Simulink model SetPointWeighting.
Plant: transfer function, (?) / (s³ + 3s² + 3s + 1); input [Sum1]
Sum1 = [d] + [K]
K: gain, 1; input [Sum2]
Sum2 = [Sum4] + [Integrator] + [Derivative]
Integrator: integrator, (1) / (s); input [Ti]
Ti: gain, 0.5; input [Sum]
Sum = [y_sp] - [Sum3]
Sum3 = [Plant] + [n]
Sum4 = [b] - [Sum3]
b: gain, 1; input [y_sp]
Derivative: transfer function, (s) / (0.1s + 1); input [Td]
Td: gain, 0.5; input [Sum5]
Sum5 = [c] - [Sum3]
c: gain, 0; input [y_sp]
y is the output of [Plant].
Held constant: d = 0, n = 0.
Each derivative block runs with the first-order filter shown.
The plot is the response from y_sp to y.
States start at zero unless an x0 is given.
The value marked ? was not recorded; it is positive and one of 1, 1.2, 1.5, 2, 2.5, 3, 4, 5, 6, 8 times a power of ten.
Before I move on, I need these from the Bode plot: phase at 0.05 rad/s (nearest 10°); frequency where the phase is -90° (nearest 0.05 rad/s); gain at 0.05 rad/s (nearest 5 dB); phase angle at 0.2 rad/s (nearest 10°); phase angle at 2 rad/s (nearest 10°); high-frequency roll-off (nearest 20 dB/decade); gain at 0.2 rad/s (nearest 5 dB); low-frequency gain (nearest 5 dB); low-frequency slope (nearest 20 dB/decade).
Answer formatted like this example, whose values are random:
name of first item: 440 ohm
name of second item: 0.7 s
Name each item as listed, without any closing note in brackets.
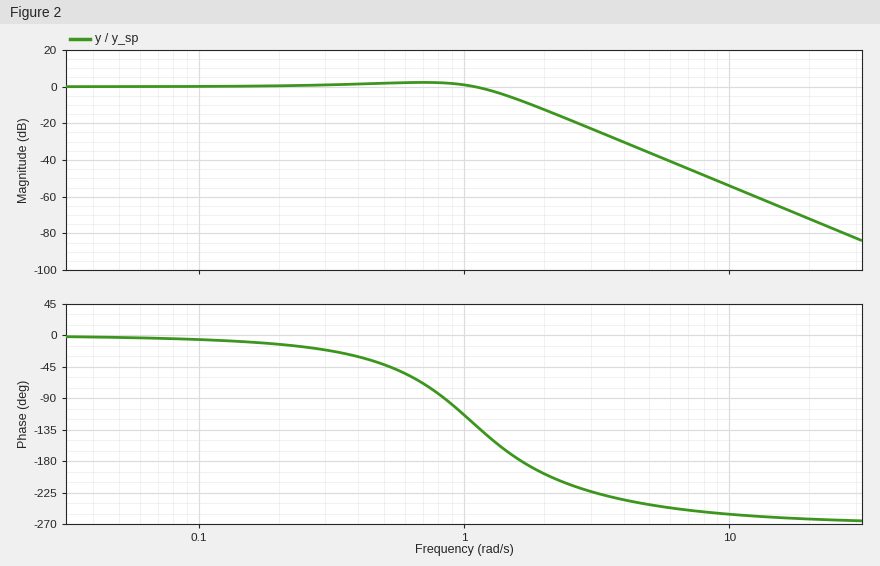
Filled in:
phase at 0.05 rad/s: 0°
frequency where the phase is -90°: 0.85 rad/s
gain at 0.05 rad/s: 0 dB
phase angle at 0.2 rad/s: -10°
phase angle at 2 rad/s: -200°
high-frequency roll-off: -60 dB/decade
gain at 0.2 rad/s: 0 dB
low-frequency gain: 0 dB
low-frequency slope: 0 dB/decade
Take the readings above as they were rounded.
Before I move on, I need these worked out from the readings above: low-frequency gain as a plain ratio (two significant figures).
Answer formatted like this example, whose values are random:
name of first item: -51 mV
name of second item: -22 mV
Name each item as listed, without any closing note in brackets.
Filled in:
low-frequency gain as a plain ratio: 1.0
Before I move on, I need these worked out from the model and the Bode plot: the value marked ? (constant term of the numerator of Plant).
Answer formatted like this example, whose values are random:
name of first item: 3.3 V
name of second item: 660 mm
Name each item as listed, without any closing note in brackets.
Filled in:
the value marked ?: 2
